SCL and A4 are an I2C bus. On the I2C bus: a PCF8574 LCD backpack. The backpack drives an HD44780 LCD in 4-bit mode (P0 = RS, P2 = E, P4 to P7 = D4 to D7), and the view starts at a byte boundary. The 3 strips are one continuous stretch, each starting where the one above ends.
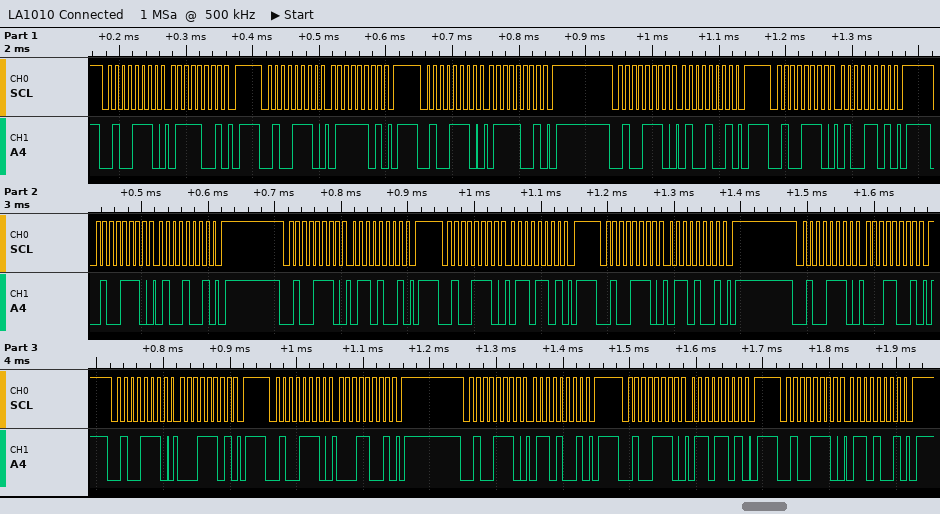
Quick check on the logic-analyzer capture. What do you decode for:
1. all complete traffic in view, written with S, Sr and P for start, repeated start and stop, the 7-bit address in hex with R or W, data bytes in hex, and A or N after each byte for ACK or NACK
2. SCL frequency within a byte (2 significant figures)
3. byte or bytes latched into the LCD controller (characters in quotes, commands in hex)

S 27W A 79 A P S 27W A 7D A P S 27W A 79 A P S 27W A 49 A P S 27W A 4D A P S 27W A 49 A P S 27W A 69 A P S 27W A 6D A P S 27W A 69 A P S 27W A 19 A P S 27W A 1D A P S 27W A 19 A P S 27W A 69 A P S 27W A 6D A P S 27W A 69 A P
100 kHz
't' 'a'
